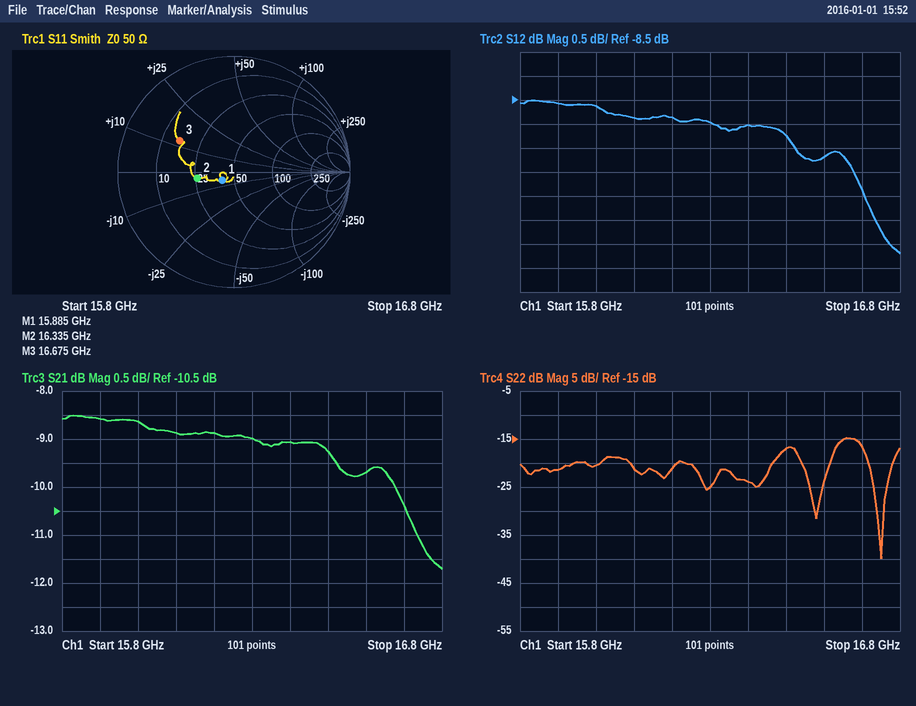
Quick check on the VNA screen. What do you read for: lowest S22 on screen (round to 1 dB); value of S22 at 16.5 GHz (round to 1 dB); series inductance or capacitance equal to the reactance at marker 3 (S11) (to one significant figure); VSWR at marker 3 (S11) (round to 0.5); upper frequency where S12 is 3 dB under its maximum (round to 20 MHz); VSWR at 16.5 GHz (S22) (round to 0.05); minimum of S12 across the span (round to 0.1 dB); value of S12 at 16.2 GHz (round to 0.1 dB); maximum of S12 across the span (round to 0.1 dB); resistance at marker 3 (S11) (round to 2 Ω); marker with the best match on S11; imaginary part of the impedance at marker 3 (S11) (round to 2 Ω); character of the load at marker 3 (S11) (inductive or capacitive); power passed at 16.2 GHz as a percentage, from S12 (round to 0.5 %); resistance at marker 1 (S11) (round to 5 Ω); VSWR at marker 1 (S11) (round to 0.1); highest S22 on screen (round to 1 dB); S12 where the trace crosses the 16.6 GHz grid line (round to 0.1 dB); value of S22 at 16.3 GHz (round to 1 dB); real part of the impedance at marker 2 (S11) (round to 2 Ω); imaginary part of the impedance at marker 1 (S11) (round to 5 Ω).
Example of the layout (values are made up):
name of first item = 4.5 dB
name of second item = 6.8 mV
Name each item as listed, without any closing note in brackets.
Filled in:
lowest S22 on screen = -40 dB
value of S22 at 16.5 GHz = -17 dB
series inductance or capacitance equal to the reactance at marker 3 (S11) = 100 pH
VSWR at marker 3 (S11) = 3.5
upper frequency where S12 is 3 dB under its maximum = 16.78 GHz
VSWR at 16.5 GHz (S22) = 1.35
minimum of S12 across the span = -11.7 dB
value of S12 at 16.2 GHz = -8.9 dB
maximum of S12 across the span = -8.5 dB
resistance at marker 3 (S11) = 16 Ω
marker with the best match on S11 = marker 1
imaginary part of the impedance at marker 3 (S11) = +12 Ω
character of the load at marker 3 (S11) = inductive
power passed at 16.2 GHz as a percentage, from S12 = 13.0 %
resistance at marker 1 (S11) = 40 Ω
VSWR at marker 1 (S11) = 1.3
highest S22 on screen = -15 dB
S12 where the trace crosses the 16.6 GHz grid line = -9.7 dB
value of S22 at 16.3 GHz = -25 dB
real part of the impedance at marker 2 (S11) = 26 Ω
imaginary part of the impedance at marker 1 (S11) = -5 Ω
